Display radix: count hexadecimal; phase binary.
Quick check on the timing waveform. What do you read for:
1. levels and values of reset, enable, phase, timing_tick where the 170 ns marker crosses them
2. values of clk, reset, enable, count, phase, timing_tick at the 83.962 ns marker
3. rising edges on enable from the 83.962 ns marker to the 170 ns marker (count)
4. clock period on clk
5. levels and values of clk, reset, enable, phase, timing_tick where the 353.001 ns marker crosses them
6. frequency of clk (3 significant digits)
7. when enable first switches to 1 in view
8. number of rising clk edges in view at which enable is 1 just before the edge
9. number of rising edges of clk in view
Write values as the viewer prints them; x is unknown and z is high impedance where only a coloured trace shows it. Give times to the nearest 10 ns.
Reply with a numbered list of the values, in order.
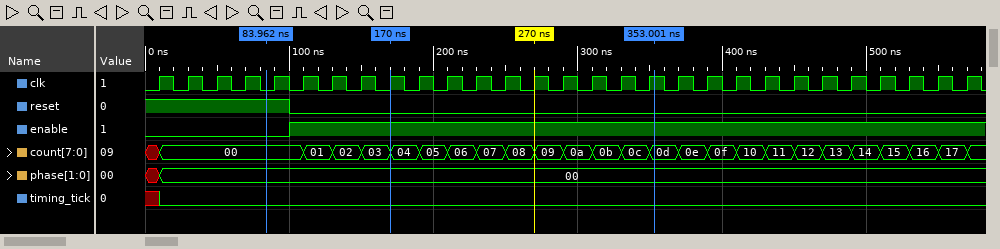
1. reset=0, enable=1, phase=00, timing_tick=0
2. clk=0, reset=1, enable=0, count=00, phase=00, timing_tick=0
3. 1
4. 20 ns
5. clk=1, reset=0, enable=1, phase=00, timing_tick=0
6. 50.0 MHz
7. 100 ns
8. 24
9. 29
